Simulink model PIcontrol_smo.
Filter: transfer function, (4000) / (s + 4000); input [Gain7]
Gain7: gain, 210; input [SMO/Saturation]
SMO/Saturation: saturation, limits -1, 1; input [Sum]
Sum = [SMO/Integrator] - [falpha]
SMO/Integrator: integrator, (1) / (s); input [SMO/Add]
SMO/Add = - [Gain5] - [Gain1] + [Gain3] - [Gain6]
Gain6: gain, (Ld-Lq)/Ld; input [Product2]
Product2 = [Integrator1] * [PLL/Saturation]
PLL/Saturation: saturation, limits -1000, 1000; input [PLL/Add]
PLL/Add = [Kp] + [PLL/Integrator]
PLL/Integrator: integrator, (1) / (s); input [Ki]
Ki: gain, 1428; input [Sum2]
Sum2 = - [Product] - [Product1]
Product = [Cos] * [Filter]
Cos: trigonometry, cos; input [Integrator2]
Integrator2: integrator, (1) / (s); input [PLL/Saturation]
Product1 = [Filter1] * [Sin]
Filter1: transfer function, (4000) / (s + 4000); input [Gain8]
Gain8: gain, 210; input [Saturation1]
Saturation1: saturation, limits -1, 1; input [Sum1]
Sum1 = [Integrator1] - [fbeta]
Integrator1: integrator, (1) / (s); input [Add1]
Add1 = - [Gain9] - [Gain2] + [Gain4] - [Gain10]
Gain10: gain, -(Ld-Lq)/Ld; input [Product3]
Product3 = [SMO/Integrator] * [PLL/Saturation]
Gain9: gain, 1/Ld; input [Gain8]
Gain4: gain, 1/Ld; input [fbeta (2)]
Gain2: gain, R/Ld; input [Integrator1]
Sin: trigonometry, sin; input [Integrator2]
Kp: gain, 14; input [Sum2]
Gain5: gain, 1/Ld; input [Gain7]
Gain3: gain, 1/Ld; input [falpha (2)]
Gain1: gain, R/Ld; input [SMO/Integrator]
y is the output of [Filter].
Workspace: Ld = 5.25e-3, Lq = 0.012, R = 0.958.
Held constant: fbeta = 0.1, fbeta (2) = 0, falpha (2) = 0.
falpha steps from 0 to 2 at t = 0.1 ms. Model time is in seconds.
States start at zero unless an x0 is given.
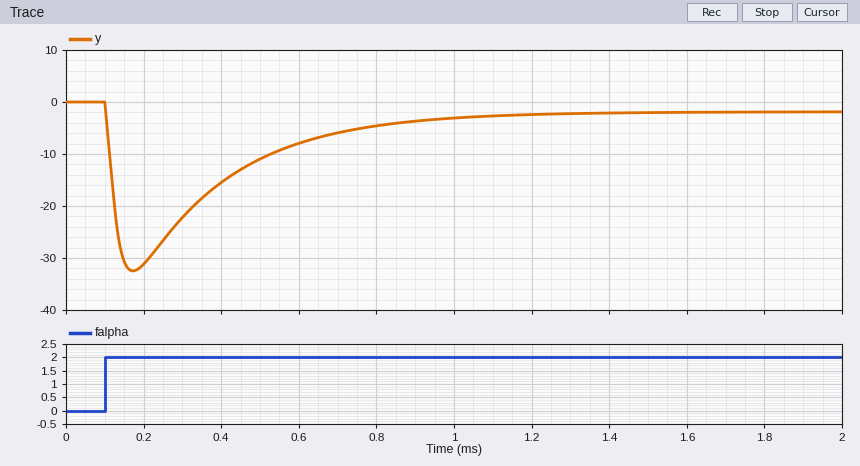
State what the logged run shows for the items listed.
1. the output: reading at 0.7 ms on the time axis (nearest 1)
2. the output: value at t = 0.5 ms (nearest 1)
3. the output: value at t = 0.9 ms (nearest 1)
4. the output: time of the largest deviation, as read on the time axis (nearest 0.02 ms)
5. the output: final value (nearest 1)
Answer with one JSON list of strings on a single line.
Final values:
["-6", "-11", "-4", "0.18 ms", "-2"]
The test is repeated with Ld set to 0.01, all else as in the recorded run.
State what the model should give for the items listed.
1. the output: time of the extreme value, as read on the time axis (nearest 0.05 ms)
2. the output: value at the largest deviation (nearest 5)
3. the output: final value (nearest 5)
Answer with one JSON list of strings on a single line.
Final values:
["0.20 ms", "-55", "0"]
